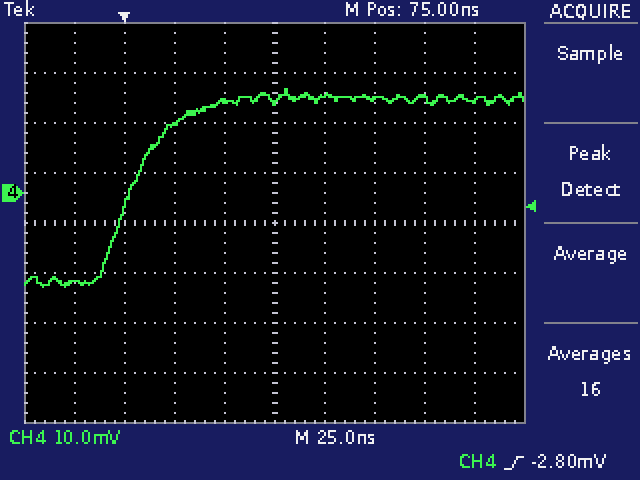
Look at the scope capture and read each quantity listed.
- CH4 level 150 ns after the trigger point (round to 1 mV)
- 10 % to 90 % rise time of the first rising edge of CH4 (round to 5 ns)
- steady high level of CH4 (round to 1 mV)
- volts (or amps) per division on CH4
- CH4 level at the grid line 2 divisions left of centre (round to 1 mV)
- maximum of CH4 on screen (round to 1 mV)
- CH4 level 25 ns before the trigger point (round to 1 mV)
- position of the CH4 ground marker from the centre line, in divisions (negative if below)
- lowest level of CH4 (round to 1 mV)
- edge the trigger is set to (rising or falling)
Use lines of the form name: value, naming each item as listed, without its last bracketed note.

CH4 level 150 ns after the trigger point: 19 mV
10 % to 90 % rise time of the first rising edge of CH4: 40 ns
steady high level of CH4: 19 mV
volts (or amps) per division on CH4: 10 mV
CH4 level at the grid line 2 divisions left of centre: 14 mV
maximum of CH4 on screen: 21 mV
CH4 level 25 ns before the trigger point: -18 mV
position of the CH4 ground marker from the centre line, in divisions: +0.6 div
lowest level of CH4: -19 mV
edge the trigger is set to: rising
